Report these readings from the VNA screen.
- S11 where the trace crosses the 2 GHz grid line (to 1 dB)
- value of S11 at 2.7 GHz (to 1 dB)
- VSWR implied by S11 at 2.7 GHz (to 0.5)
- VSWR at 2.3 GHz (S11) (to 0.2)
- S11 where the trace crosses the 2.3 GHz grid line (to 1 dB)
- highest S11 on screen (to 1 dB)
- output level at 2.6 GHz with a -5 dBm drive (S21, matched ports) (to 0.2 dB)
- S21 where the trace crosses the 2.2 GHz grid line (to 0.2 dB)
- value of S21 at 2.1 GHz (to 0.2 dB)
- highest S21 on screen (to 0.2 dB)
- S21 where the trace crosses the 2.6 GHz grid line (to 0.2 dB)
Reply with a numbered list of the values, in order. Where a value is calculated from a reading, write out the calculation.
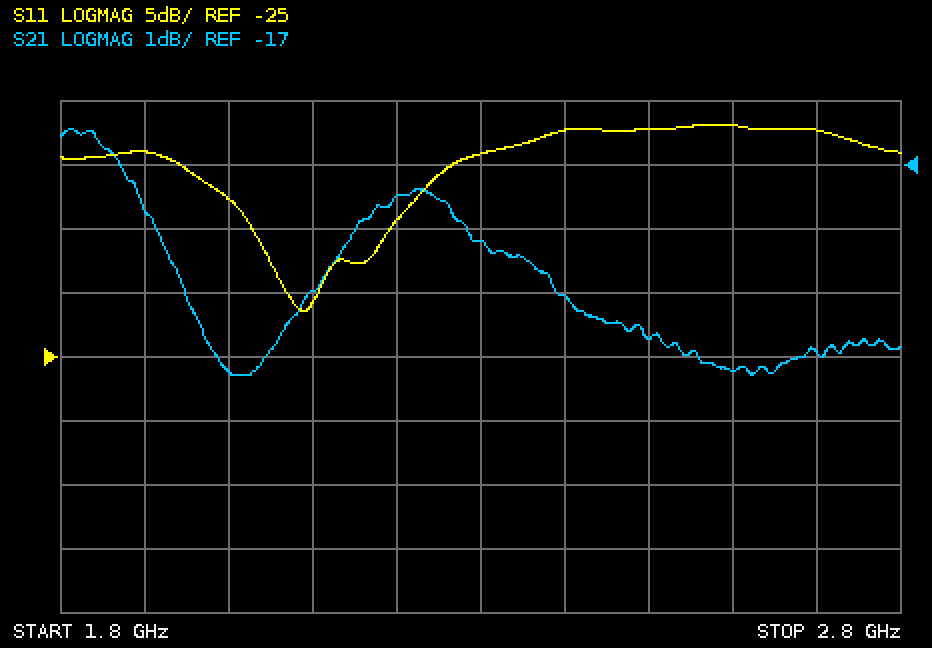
1. -13 dB
2. -7 dB
3. |Γ| = 10^(-7/20) = 0.4467; VSWR = (1 + 0.4467)/(1 − 0.4467) ≈ 2.61, so 2.5 to the nearest 0.5
4. |Γ| = 10^(-9/20) = 0.3548; VSWR = (1 + 0.3548)/(1 − 0.3548) ≈ 2.10, so 2.0 to the nearest 0.2
5. -9 dB
6. -7 dB
7. -5 dBm + (-20.2 dB) = -25.2 dBm
8. -17.4 dB
9. -19.0 dB
10. -16.4 dB
11. -20.2 dB
